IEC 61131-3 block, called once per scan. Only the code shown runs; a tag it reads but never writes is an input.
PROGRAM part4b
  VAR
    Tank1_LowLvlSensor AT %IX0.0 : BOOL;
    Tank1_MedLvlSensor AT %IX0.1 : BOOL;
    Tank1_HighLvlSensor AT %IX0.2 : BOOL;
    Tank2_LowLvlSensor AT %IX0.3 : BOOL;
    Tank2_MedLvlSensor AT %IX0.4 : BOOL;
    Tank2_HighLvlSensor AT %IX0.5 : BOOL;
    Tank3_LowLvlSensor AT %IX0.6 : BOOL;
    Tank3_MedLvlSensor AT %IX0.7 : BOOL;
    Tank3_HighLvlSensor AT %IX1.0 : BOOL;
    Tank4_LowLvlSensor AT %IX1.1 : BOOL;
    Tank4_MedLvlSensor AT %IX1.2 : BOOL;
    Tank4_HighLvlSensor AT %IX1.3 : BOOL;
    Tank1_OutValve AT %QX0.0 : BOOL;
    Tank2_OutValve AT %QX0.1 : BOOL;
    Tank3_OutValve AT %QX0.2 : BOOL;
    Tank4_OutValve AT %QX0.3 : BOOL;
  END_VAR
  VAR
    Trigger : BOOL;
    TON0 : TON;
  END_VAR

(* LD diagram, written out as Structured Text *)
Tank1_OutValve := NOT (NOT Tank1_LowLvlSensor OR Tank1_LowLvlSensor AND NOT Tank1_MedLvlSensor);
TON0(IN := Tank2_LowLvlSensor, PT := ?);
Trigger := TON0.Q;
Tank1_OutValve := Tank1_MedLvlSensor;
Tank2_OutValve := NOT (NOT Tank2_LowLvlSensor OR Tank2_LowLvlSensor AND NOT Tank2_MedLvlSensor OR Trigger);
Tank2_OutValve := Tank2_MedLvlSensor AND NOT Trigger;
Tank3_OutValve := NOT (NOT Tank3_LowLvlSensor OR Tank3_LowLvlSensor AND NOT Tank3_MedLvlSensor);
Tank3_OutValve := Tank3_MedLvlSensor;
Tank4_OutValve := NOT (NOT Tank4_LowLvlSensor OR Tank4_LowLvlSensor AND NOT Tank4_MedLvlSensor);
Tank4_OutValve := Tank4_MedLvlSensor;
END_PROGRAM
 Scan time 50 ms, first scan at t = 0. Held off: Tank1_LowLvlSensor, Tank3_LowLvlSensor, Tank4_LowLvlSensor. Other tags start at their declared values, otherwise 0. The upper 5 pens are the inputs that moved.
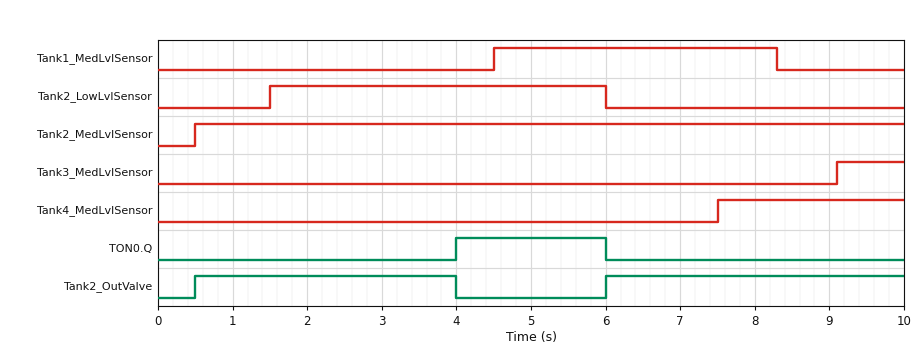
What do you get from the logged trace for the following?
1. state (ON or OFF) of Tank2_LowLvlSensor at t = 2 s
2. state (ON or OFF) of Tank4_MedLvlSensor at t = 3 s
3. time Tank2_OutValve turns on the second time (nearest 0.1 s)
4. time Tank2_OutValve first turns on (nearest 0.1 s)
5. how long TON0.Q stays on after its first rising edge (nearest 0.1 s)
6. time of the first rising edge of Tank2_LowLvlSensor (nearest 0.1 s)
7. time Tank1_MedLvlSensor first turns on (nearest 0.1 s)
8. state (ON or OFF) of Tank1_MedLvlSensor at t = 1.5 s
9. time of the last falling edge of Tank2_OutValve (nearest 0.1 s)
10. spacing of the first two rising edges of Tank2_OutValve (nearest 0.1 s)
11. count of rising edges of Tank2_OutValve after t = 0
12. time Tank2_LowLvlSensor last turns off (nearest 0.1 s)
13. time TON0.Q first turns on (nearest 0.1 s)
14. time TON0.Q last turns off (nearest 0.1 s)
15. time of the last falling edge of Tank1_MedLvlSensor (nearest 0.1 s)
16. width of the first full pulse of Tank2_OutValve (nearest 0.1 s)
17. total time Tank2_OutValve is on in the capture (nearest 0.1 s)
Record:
ON
OFF
6.0 s
0.5 s
2.0 s
1.5 s
4.5 s
OFF
4.0 s
5.5 s
2
6.0 s
4.0 s
6.0 s
8.3 s
3.5 s
7.5 s
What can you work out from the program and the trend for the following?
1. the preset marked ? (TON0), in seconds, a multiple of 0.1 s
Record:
2.5 s
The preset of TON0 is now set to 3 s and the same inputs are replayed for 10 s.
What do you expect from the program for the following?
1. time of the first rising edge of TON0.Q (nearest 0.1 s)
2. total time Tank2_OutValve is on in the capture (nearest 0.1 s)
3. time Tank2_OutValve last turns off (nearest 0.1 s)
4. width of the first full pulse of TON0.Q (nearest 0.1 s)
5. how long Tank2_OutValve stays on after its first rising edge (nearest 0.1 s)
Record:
4.5 s
8.0 s
4.5 s
1.5 s
4.0 s
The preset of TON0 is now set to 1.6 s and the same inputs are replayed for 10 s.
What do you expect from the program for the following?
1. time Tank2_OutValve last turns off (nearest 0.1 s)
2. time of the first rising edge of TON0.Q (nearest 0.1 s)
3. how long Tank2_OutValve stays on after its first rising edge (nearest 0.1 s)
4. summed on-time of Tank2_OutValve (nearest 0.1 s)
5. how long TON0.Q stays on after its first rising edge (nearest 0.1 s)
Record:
3.1 s
3.1 s
2.6 s
6.6 s
2.9 s
